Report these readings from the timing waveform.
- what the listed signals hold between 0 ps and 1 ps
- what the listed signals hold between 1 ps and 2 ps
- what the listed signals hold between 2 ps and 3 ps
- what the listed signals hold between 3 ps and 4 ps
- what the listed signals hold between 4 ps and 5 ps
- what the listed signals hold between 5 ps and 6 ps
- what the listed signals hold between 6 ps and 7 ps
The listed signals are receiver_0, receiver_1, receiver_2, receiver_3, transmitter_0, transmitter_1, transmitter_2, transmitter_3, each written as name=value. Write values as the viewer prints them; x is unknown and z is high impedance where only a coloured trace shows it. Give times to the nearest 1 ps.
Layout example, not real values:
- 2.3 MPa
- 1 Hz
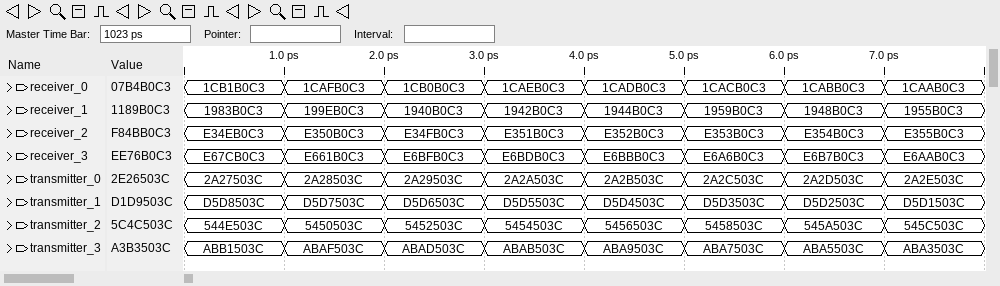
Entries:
- receiver_0=1CB1B0C3, receiver_1=1983B0C3, receiver_2=E34EB0C3, receiver_3=E67CB0C3, transmitter_0=2A27503C, transmitter_1=D5D8503C, transmitter_2=544E503C, transmitter_3=ABB1503C
- receiver_0=1CAFB0C3, receiver_1=199EB0C3, receiver_2=E350B0C3, receiver_3=E661B0C3, transmitter_0=2A28503C, transmitter_1=D5D7503C, transmitter_2=5450503C, transmitter_3=ABAF503C
- receiver_0=1CB0B0C3, receiver_1=1940B0C3, receiver_2=E34FB0C3, receiver_3=E6BFB0C3, transmitter_0=2A29503C, transmitter_1=D5D6503C, transmitter_2=5452503C, transmitter_3=ABAD503C
- receiver_0=1CAEB0C3, receiver_1=1942B0C3, receiver_2=E351B0C3, receiver_3=E6BDB0C3, transmitter_0=2A2A503C, transmitter_1=D5D5503C, transmitter_2=5454503C, transmitter_3=ABAB503C
- receiver_0=1CADB0C3, receiver_1=1944B0C3, receiver_2=E352B0C3, receiver_3=E6BBB0C3, transmitter_0=2A2B503C, transmitter_1=D5D4503C, transmitter_2=5456503C, transmitter_3=ABA9503C
- receiver_0=1CACB0C3, receiver_1=1959B0C3, receiver_2=E353B0C3, receiver_3=E6A6B0C3, transmitter_0=2A2C503C, transmitter_1=D5D3503C, transmitter_2=5458503C, transmitter_3=ABA7503C
- receiver_0=1CABB0C3, receiver_1=1948B0C3, receiver_2=E354B0C3, receiver_3=E6B7B0C3, transmitter_0=2A2D503C, transmitter_1=D5D2503C, transmitter_2=545A503C, transmitter_3=ABA5503C
